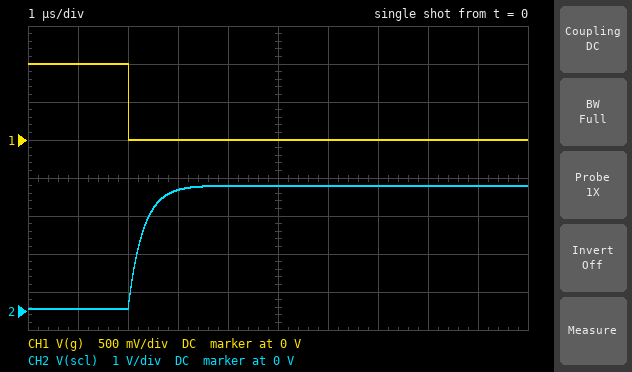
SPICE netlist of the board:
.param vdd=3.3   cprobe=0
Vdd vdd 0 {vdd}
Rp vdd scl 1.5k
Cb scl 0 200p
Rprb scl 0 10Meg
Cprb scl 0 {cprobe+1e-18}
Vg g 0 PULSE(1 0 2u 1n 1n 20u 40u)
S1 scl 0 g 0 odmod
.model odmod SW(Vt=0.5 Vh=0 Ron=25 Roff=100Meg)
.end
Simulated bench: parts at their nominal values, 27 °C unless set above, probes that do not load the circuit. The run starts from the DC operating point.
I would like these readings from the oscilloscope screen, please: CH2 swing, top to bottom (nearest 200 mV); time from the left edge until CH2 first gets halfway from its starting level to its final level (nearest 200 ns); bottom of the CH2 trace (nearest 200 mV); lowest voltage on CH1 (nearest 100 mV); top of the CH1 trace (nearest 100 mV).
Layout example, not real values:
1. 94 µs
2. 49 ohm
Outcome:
1. 3.2 V
2. 2.2 µs
3. 0 V
4. 0 V
5. 1.0 V
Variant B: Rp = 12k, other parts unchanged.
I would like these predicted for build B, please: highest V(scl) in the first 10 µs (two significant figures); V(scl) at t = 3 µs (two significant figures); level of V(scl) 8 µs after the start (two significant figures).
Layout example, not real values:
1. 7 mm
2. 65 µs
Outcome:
1. 3.2 V
2. 1.1 V
3. 3.0 V
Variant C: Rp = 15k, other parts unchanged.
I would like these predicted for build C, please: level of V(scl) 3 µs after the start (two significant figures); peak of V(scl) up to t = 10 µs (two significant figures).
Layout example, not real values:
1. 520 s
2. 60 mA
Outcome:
1. 940 mV
2. 3.1 V
